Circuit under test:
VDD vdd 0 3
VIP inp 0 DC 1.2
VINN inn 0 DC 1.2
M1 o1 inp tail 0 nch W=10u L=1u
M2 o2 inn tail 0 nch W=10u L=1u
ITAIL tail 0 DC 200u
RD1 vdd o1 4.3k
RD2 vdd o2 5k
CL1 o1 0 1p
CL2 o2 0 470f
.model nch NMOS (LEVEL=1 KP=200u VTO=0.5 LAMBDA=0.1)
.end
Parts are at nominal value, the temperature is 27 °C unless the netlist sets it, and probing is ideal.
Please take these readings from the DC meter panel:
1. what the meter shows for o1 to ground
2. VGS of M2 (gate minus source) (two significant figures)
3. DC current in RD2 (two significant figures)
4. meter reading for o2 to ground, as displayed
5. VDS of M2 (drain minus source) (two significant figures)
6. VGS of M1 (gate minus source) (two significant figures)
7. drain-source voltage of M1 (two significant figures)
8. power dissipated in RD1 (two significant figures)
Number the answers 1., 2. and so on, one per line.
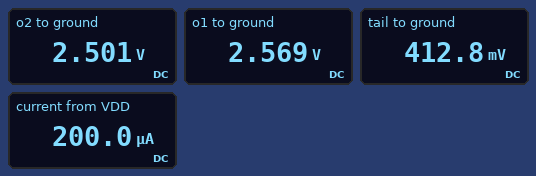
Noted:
1. 2.569 V
2. 790 mV
3. 100 µA
4. 2.501 V
5. 2.1 V
6. 790 mV
7. 2.2 V
8. 43 µW
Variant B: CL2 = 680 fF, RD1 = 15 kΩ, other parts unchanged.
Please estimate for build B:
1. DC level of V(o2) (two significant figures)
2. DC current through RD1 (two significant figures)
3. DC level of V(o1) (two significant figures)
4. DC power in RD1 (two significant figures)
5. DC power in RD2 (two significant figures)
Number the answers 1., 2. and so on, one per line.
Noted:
1. 2.5 V
2. 96 µA
3. 1.6 V
4. 140 µW
5. 54 µW
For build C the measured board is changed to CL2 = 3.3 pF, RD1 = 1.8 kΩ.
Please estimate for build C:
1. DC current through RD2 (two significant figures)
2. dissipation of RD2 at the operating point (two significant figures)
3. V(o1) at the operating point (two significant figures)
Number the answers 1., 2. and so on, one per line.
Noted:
1. 99 µA
2. 49 µW
3. 2.8 V
